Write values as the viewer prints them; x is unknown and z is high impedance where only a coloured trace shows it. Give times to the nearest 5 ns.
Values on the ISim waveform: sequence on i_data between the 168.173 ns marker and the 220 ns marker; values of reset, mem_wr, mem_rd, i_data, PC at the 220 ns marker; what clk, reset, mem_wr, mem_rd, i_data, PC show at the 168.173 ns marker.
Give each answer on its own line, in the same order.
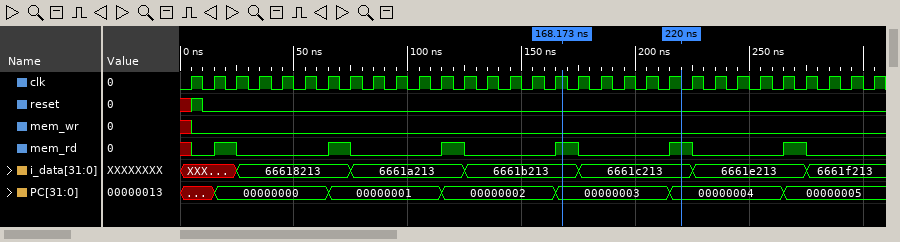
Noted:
6661b213, 6661c213
reset=0, mem_wr=0, mem_rd=1, i_data=6661c213, PC=00000004
clk=1, reset=0, mem_wr=0, mem_rd=1, i_data=6661b213, PC=00000003
